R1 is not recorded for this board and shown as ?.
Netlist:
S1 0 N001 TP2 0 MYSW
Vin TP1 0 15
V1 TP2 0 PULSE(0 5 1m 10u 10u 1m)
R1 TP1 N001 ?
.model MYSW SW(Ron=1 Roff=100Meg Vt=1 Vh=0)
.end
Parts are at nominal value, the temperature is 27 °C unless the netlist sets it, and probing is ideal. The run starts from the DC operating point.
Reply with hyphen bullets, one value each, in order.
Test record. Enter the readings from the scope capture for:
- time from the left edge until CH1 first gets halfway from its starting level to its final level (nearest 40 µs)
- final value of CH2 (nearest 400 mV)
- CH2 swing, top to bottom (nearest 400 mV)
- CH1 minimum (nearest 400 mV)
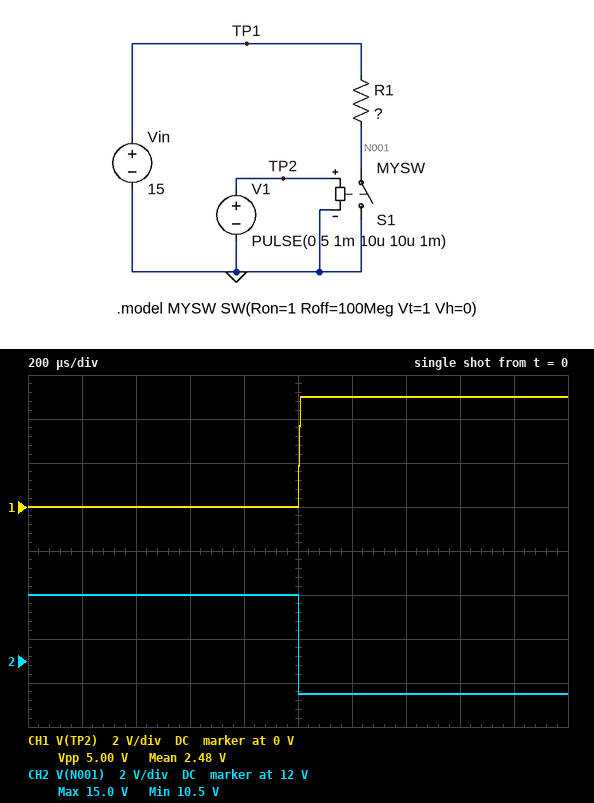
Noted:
- 1.00 ms
- 10.4 V
- 4.4 V
- 0 V
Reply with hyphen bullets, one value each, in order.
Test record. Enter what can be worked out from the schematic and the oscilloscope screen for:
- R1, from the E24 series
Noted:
- 0.43 Ω
